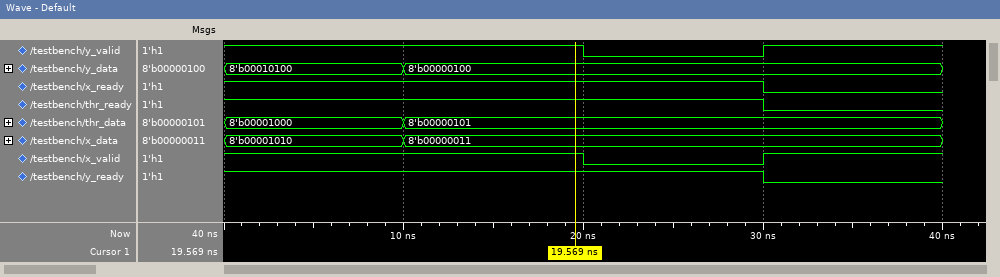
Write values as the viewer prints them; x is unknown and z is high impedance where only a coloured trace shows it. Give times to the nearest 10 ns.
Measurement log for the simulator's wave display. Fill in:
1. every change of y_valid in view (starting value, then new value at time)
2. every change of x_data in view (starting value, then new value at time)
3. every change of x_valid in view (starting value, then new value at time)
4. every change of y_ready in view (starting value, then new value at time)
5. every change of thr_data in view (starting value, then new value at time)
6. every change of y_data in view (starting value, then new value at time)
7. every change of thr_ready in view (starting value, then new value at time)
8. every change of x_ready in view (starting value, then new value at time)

1, 0 at 20 ns, 1 at 30 ns
8'b00001010, 8'b00000011 at 10 ns
1, 0 at 20 ns, 1 at 30 ns
1, 0 at 30 ns
8'b00001000, 8'b00000101 at 10 ns
8'b00010100, 8'b00000100 at 10 ns
1, 0 at 30 ns
1, 0 at 30 ns
